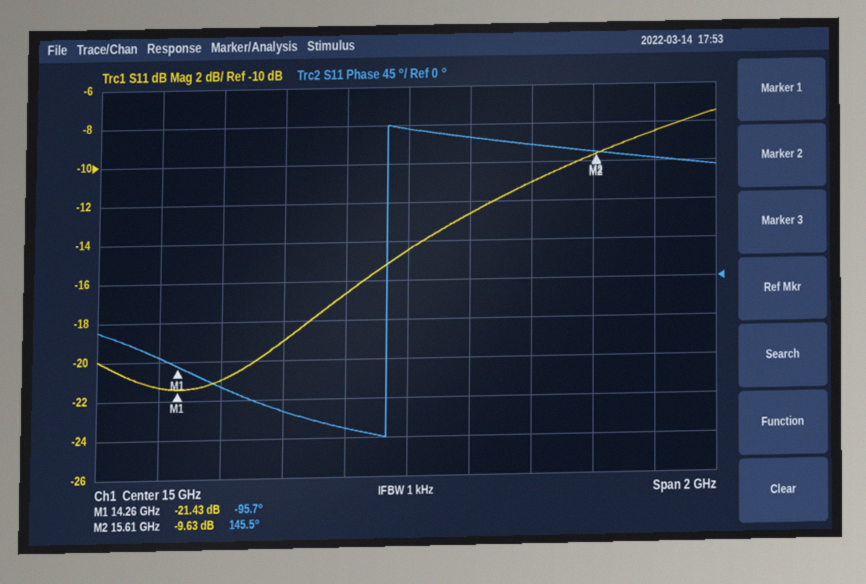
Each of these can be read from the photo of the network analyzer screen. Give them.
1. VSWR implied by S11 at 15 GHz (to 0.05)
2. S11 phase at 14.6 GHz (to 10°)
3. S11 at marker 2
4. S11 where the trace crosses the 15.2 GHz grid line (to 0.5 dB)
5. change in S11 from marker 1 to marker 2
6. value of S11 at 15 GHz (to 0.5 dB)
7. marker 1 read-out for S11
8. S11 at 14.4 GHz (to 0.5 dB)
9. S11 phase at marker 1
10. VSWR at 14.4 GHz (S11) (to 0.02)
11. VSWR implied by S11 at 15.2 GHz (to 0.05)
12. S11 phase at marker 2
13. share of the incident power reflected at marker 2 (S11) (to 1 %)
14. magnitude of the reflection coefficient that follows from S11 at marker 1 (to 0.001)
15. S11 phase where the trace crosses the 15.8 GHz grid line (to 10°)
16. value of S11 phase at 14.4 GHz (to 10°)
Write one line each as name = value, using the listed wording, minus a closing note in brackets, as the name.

VSWR implied by S11 at 15 GHz = 1.45
S11 phase at 14.6 GHz = -150°
S11 at marker 2 = -9.63 dB
S11 where the trace crosses the 15.2 GHz grid line = -12.5 dB
change in S11 from marker 1 to marker 2 = 11.80 dB
value of S11 at 15 GHz = -14.5 dB
marker 1 read-out for S11 = -21.43 dB
S11 at 14.4 GHz = -21.0 dB
S11 phase at marker 1 = -95.7°
VSWR at 14.4 GHz (S11) = 1.20
VSWR implied by S11 at 15.2 GHz = 1.60
S11 phase at marker 2 = 145.5°
share of the incident power reflected at marker 2 (S11) = 11 %
magnitude of the reflection coefficient that follows from S11 at marker 1 = 0.085
S11 phase where the trace crosses the 15.8 GHz grid line = 140°
value of S11 phase at 14.4 GHz = -120°
